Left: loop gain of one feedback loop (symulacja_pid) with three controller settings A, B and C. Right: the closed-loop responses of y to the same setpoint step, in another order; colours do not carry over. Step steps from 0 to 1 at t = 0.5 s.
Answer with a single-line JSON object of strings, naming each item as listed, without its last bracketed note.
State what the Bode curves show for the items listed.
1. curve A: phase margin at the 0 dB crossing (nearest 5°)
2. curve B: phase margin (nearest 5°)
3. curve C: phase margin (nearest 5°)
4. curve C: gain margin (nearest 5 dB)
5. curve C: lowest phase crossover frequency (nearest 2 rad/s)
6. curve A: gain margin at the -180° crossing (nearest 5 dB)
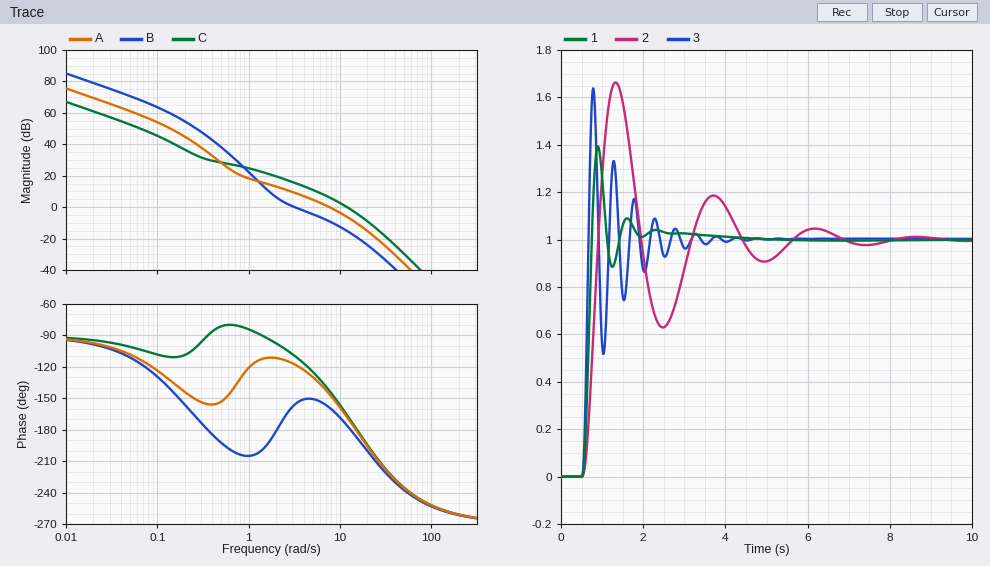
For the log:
{"curve A: phase margin at the 0 dB crossing": "35°", "curve B: phase margin": "25°", "curve C: phase margin": "15°", "curve C: gain margin": "5 dB", "curve C: lowest phase crossover frequency": "16 rad/s", "curve A: gain margin at the -180° crossing": "10 dB"}
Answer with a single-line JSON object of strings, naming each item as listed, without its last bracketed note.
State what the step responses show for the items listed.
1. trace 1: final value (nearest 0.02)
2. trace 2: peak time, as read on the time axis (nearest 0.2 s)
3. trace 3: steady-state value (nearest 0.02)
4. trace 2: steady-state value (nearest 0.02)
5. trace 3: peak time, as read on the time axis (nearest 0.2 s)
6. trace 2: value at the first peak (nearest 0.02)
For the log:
{"trace 1: final value": "1.00", "trace 2: peak time, as read on the time axis": "1.4 s", "trace 3: steady-state value": "1.00", "trace 2: steady-state value": "1.00", "trace 3: peak time, as read on the time axis": "0.8 s", "trace 2: value at the first peak": "1.66"}
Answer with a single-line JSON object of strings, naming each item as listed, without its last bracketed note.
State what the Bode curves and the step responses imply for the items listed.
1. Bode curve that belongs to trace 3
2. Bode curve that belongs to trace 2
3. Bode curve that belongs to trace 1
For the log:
{"Bode curve that belongs to trace 3": "C", "Bode curve that belongs to trace 2": "B", "Bode curve that belongs to trace 1": "A"}
